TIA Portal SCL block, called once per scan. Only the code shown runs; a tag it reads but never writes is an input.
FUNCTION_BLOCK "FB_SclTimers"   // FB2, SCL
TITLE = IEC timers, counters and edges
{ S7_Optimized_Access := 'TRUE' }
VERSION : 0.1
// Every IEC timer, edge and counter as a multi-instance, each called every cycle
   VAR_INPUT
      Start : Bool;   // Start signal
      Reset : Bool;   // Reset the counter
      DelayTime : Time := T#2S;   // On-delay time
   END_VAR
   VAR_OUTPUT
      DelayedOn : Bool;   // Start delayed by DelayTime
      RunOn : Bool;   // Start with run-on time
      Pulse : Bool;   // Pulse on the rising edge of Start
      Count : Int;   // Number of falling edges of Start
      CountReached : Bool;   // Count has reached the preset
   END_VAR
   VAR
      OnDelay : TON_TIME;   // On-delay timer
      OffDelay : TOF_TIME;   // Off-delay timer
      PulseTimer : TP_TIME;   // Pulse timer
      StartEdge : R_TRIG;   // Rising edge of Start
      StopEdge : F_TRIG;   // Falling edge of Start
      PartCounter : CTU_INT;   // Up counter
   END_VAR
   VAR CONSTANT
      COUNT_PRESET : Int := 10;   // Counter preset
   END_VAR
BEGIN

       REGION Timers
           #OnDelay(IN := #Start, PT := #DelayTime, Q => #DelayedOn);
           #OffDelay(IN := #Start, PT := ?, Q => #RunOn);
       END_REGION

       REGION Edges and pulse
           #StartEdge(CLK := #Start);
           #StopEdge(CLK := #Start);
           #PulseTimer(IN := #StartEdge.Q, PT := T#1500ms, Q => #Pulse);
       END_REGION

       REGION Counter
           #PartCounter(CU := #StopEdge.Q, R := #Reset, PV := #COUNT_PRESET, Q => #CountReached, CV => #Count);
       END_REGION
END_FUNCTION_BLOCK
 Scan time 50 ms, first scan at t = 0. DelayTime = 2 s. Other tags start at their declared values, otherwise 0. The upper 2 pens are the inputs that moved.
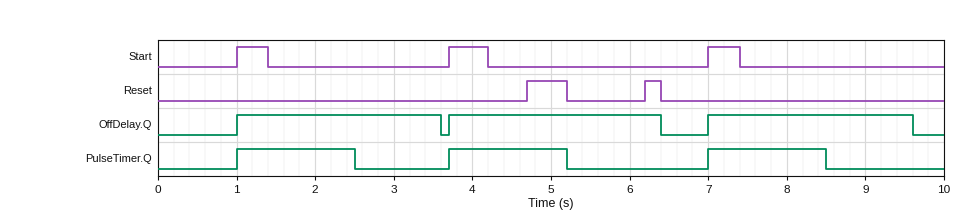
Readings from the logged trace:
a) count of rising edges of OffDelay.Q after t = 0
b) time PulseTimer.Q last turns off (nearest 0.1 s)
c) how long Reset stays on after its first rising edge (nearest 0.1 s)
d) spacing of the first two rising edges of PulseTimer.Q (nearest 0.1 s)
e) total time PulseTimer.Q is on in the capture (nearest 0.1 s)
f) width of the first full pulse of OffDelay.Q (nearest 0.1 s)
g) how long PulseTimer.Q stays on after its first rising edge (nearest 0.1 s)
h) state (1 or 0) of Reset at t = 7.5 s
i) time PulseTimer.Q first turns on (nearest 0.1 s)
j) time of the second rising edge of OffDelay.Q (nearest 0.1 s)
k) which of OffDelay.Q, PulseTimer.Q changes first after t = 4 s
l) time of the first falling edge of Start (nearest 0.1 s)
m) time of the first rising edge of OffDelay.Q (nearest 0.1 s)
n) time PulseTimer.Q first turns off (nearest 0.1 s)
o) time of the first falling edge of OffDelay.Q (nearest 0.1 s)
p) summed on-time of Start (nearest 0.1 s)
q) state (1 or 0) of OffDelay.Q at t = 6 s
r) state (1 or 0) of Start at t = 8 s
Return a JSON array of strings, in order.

["3", "8.5 s", "0.5 s", "2.7 s", "4.5 s", "2.6 s", "1.5 s", "0", "1.0 s", "3.7 s", "PulseTimer.Q", "1.4 s", "1.0 s", "2.5 s", "3.6 s", "1.3 s", "1", "0"]
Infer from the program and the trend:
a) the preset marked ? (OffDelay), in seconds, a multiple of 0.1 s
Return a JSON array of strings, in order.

["2.2 s"]
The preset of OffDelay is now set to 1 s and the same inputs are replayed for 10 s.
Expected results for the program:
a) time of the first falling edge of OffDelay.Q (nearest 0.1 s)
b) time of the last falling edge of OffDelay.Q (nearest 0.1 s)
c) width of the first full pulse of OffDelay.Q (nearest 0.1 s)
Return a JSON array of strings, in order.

["2.4 s", "8.4 s", "1.4 s"]
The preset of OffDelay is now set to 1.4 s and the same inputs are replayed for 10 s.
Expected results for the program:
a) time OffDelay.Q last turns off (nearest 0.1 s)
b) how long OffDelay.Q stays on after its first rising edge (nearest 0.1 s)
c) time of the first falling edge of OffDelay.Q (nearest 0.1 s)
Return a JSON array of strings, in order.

["8.8 s", "1.8 s", "2.8 s"]
